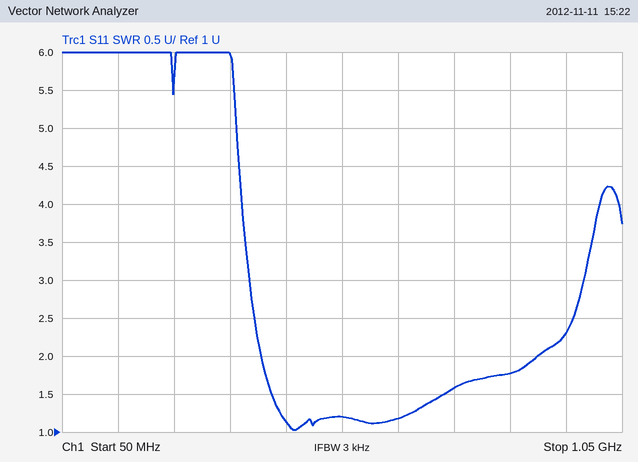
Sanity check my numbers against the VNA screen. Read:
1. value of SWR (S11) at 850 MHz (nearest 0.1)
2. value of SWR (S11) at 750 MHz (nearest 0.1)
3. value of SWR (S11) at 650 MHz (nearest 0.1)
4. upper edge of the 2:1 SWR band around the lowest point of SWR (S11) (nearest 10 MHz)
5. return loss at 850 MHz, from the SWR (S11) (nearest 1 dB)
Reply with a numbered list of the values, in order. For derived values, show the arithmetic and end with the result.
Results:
1. 1.8
2. 1.6
3. 1.2
4. 900 MHz
5. −20 log10((1.8 − 1)/(1.8 + 1)) ≈ 11 dB
